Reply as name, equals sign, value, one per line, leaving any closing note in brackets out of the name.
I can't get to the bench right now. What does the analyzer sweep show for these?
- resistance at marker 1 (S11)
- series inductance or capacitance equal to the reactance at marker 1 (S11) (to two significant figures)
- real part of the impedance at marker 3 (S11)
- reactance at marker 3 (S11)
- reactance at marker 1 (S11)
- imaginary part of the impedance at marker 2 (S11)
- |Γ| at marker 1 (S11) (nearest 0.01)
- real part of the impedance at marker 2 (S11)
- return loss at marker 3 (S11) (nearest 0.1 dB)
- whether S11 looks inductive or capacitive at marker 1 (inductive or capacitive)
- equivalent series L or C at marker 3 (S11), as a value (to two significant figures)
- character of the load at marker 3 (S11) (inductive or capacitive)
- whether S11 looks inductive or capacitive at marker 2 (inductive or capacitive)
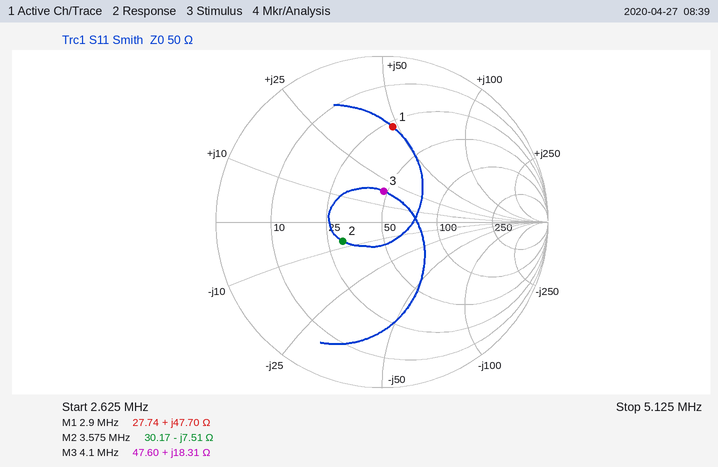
resistance at marker 1 = 27.74 Ω
series inductance or capacitance equal to the reactance at marker 1 (S11) = 2.6 µH
real part of the impedance at marker 3 = 47.60 Ω
reactance at marker 3 = +18.31 Ω
reactance at marker 1 = +47.70 Ω
imaginary part of the impedance at marker 2 = -7.51 Ω
|Γ| at marker 1 (S11) = 0.58
real part of the impedance at marker 2 = 30.17 Ω
return loss at marker 3 (S11) = 14.6 dB
whether S11 looks inductive or capacitive at marker 1 = inductive
equivalent series L or C at marker 3 (S11), as a value = 710 nH
character of the load at marker 3 (S11) = inductive
whether S11 looks inductive or capacitive at marker 2 = capacitive
